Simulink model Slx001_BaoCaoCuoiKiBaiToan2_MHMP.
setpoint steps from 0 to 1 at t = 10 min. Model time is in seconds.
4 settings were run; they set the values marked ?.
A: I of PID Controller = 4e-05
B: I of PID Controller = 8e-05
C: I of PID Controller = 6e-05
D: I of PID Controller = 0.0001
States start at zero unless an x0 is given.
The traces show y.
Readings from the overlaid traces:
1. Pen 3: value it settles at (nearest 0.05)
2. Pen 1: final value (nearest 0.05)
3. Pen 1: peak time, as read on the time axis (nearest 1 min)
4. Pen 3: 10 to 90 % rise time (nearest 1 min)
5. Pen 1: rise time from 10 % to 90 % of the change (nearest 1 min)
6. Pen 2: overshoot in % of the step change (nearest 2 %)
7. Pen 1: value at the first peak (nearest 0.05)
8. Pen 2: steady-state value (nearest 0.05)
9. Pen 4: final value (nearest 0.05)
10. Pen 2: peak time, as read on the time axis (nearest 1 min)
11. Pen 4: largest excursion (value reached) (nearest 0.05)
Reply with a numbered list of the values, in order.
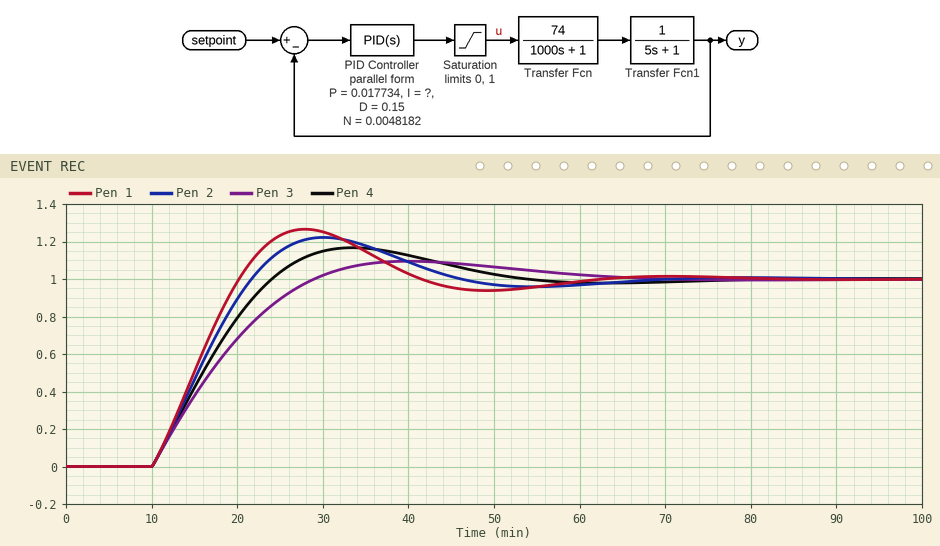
1. 1.00
2. 1.00
3. 28 min
4. 14 min
5. 8 min
6. 22 %
7. 1.25
8. 1.00
9. 1.00
10. 30 min
11. 1.15
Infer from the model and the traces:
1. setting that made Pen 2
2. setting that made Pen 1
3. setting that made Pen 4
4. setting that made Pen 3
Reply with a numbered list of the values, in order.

1. B
2. D
3. C
4. A
